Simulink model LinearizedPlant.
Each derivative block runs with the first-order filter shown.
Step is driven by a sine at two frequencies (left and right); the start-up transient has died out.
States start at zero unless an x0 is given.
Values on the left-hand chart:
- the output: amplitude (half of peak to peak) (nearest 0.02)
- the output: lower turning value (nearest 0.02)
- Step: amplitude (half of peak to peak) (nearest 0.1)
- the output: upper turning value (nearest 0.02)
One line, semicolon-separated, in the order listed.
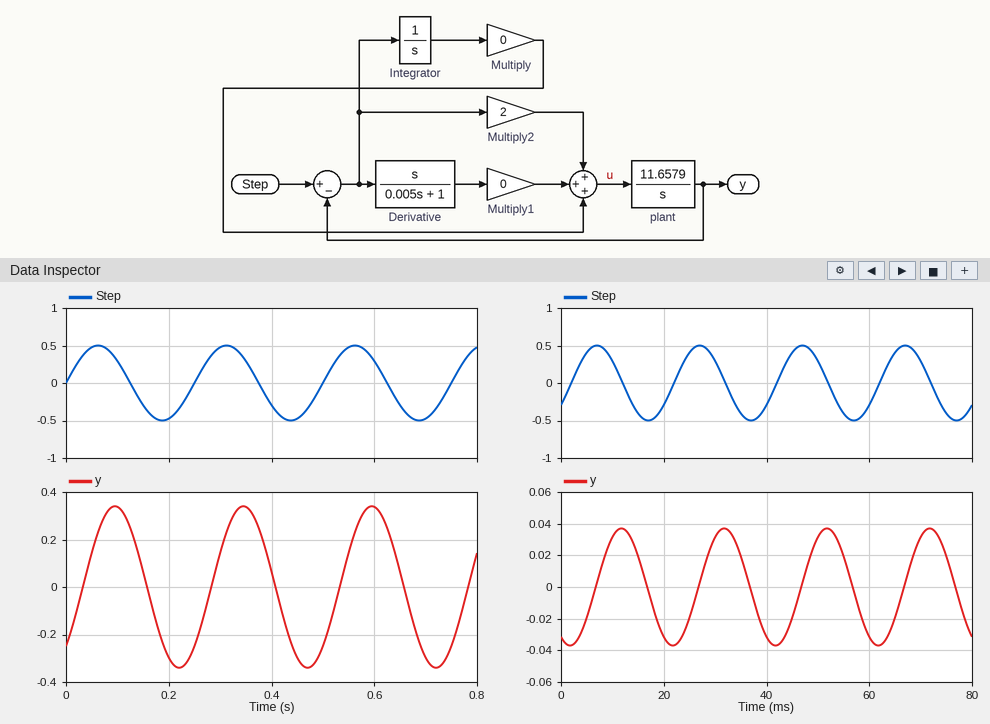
0.34; -0.34; 0.5; 0.34
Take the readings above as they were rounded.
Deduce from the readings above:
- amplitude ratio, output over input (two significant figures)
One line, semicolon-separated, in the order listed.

0.68
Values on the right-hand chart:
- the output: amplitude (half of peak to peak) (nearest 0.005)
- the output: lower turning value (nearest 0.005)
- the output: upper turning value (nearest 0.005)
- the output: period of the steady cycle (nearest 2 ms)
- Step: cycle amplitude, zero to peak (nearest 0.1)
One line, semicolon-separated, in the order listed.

0.035; -0.035; 0.035; 20 ms; 0.5
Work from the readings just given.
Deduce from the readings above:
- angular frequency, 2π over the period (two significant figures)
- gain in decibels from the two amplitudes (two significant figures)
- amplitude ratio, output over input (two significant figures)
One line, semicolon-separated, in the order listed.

0.31 rad/ms; -23 dB; 0.070
